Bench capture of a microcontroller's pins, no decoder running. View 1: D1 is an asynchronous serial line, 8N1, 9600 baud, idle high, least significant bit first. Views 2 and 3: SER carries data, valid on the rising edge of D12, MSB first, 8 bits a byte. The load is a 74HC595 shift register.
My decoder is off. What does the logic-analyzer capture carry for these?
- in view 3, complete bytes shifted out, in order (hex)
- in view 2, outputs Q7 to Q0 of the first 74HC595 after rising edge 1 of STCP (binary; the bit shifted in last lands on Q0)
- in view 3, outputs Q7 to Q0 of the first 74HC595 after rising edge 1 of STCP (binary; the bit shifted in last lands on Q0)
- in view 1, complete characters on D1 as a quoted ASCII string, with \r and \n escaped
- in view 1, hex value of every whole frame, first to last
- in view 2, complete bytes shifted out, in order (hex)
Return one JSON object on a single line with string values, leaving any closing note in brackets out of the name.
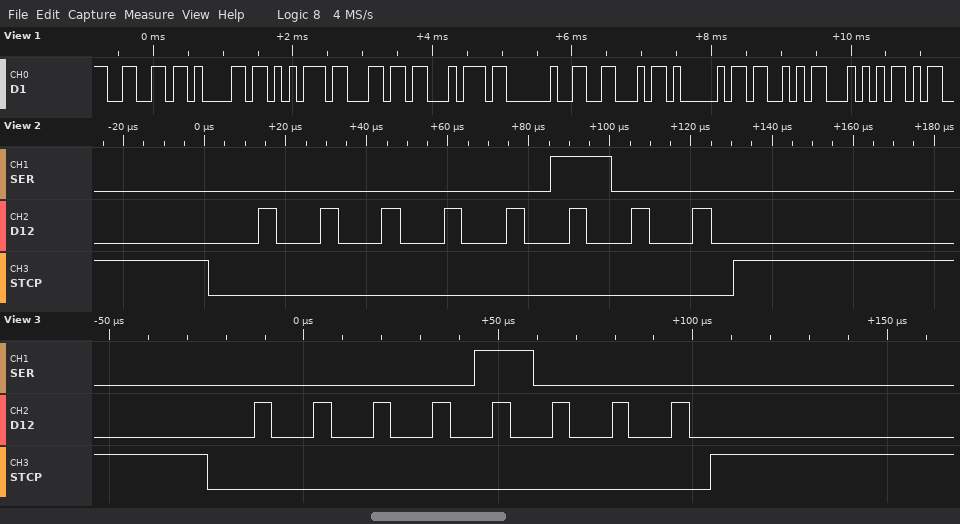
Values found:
{"in view 3, complete bytes shifted out, in order": "08", "in view 2, outputs Q7 to Q0 of the first 74HC595 after rising edge 1 of STCP": "00000100", "in view 3, outputs Q7 to Q0 of the first 74HC595 after rising edge 1 of STCP": "00001000", "in view 1, complete characters on D1 as a quoted ASCII string, with \\r and \\n escaped": "\"fault FAST\"", "in view 1, hex value of every whole frame, first to last": "0x66 0x61 0x75 0x6C 0x74 0x20 0x46 0x41 0x53 0x54", "in view 2, complete bytes shifted out, in order": "0x04"}
